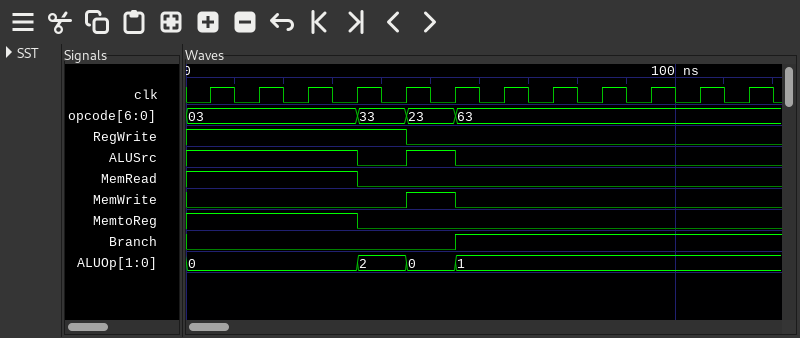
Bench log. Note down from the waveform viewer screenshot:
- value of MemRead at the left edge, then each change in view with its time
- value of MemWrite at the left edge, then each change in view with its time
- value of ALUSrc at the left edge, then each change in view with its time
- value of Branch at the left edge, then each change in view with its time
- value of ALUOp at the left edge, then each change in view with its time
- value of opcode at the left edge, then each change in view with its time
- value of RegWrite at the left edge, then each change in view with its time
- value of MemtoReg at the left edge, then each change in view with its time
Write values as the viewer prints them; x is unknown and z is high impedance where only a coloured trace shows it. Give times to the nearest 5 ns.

1, 0 at 35 ns
0, 1 at 45 ns, 0 at 55 ns
1, 0 at 35 ns, 1 at 45 ns, 0 at 55 ns
0, 1 at 55 ns
0, 2 at 35 ns, 0 at 45 ns, 1 at 55 ns
03, 33 at 35 ns, 23 at 45 ns, 63 at 55 ns
1, 0 at 45 ns
1, 0 at 35 ns
